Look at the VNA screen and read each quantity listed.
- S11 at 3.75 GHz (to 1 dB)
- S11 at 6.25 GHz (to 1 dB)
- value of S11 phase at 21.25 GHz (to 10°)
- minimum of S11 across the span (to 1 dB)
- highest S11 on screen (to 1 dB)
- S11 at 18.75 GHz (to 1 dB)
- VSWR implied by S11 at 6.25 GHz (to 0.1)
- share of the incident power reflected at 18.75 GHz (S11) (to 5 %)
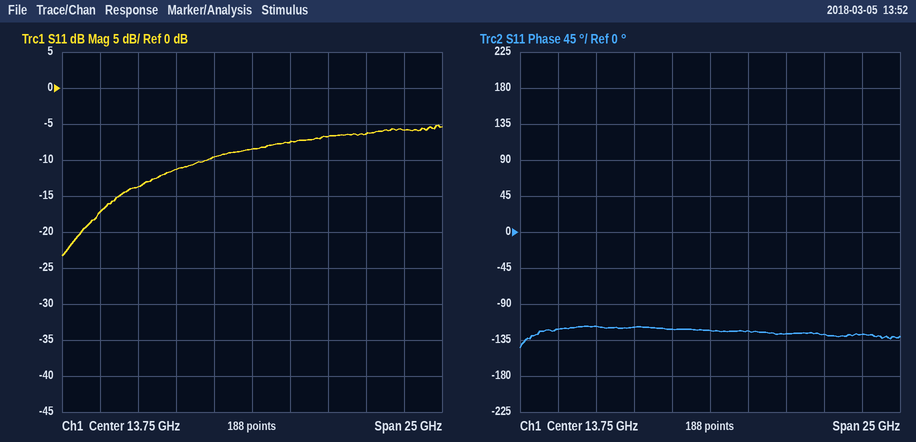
-17 dB
-14 dB
-130°
-23 dB
-5 dB
-7 dB
1.5
20 %
